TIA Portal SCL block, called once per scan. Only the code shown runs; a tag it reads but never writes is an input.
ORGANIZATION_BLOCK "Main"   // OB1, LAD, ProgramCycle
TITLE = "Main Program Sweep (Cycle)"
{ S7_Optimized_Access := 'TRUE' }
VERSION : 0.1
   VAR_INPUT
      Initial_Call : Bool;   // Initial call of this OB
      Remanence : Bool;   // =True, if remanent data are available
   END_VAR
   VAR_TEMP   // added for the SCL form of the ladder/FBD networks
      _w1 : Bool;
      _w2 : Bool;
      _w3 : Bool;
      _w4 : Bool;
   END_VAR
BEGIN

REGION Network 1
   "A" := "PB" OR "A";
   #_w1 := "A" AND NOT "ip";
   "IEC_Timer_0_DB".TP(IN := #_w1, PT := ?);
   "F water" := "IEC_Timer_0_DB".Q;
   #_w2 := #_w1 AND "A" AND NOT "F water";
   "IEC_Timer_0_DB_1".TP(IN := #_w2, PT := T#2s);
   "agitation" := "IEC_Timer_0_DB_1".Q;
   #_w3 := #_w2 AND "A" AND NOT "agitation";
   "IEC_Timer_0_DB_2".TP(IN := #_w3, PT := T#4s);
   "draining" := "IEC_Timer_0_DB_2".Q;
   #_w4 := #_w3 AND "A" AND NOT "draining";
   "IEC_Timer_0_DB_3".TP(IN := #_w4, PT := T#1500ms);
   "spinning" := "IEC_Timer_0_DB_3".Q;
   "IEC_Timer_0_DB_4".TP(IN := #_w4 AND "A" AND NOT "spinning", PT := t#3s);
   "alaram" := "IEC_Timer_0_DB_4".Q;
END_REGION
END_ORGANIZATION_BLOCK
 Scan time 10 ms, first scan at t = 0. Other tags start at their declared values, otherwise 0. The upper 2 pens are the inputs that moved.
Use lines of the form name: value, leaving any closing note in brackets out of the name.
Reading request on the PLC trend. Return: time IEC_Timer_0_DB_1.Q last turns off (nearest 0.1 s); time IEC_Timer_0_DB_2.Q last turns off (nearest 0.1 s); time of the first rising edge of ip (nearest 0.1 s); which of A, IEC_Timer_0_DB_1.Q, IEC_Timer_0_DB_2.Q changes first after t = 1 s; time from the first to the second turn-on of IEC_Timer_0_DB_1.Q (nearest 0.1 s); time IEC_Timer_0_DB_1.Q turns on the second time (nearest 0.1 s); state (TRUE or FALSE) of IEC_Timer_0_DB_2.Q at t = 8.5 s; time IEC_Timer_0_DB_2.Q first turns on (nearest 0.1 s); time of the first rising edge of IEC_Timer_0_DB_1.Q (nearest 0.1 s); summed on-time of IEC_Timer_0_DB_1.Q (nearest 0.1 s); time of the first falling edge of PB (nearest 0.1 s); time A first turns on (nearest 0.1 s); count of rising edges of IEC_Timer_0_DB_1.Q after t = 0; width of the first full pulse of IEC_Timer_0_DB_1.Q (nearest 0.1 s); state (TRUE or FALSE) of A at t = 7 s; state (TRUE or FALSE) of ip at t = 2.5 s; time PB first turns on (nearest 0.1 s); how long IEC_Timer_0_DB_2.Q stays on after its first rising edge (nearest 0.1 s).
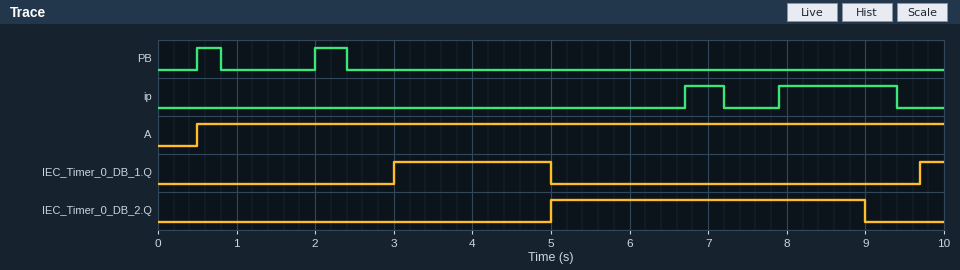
time IEC_Timer_0_DB_1.Q last turns off: 5.0 s
time IEC_Timer_0_DB_2.Q last turns off: 9.0 s
time of the first rising edge of ip: 6.7 s
which of A, IEC_Timer_0_DB_1.Q, IEC_Timer_0_DB_2.Q changes first after t = 1 s: IEC_Timer_0_DB_1.Q
time from the first to the second turn-on of IEC_Timer_0_DB_1.Q: 6.7 s
time IEC_Timer_0_DB_1.Q turns on the second time: 9.7 s
state (TRUE or FALSE) of IEC_Timer_0_DB_2.Q at t = 8.5 s: TRUE
time IEC_Timer_0_DB_2.Q first turns on: 5.0 s
time of the first rising edge of IEC_Timer_0_DB_1.Q: 3.0 s
summed on-time of IEC_Timer_0_DB_1.Q: 2.3 s
time of the first falling edge of PB: 0.8 s
time A first turns on: 0.5 s
count of rising edges of IEC_Timer_0_DB_1.Q after t = 0: 2
width of the first full pulse of IEC_Timer_0_DB_1.Q: 2.0 s
state (TRUE or FALSE) of A at t = 7 s: TRUE
state (TRUE or FALSE) of ip at t = 2.5 s: FALSE
time PB first turns on: 0.5 s
how long IEC_Timer_0_DB_2.Q stays on after its first rising edge: 4.0 s
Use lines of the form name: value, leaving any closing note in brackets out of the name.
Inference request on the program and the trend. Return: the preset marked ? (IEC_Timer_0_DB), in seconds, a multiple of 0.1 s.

the preset marked ? (IEC_Timer_0_DB), in seconds, a multiple of 0.1 s: 2.5 s
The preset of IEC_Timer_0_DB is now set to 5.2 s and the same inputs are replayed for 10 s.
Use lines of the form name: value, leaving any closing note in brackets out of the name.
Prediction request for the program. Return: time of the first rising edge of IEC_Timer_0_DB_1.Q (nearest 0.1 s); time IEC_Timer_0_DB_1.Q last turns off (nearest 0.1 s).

time of the first rising edge of IEC_Timer_0_DB_1.Q: 5.7 s
time IEC_Timer_0_DB_1.Q last turns off: 7.7 s
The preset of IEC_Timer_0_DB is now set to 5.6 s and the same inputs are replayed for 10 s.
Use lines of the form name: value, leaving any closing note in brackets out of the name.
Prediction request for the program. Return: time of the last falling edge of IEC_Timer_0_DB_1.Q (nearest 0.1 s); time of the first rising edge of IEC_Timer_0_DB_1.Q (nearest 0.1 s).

time of the last falling edge of IEC_Timer_0_DB_1.Q: 8.1 s
time of the first rising edge of IEC_Timer_0_DB_1.Q: 6.1 s
